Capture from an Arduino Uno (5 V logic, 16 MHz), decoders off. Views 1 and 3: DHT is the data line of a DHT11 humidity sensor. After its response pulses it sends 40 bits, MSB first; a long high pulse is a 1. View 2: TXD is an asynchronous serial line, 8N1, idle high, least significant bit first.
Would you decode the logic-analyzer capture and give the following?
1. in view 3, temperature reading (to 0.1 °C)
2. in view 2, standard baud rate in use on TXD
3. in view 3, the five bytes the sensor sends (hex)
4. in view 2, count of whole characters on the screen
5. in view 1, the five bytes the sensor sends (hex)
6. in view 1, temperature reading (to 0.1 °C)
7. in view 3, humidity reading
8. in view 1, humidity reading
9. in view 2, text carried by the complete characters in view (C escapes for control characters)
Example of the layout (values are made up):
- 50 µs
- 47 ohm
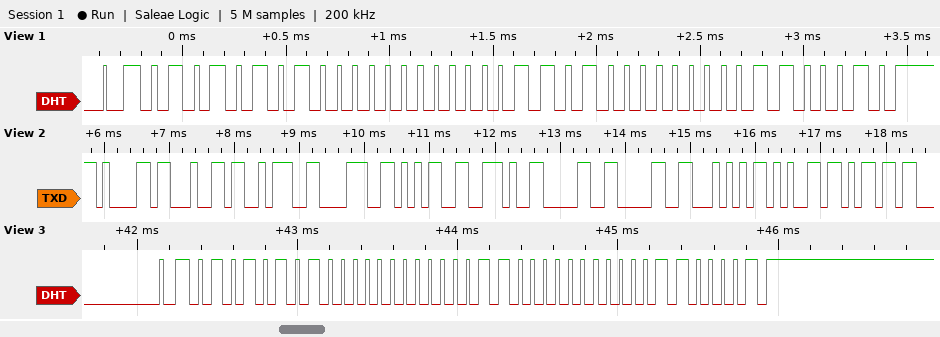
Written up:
- 12.0 °C
- 9600 baud
- 55 00 0C 00 61
- 11
- 55 00 0D 00 62
- 13.0 °C
- 85 %
- 85 %
- "ad:85.00Tem"
